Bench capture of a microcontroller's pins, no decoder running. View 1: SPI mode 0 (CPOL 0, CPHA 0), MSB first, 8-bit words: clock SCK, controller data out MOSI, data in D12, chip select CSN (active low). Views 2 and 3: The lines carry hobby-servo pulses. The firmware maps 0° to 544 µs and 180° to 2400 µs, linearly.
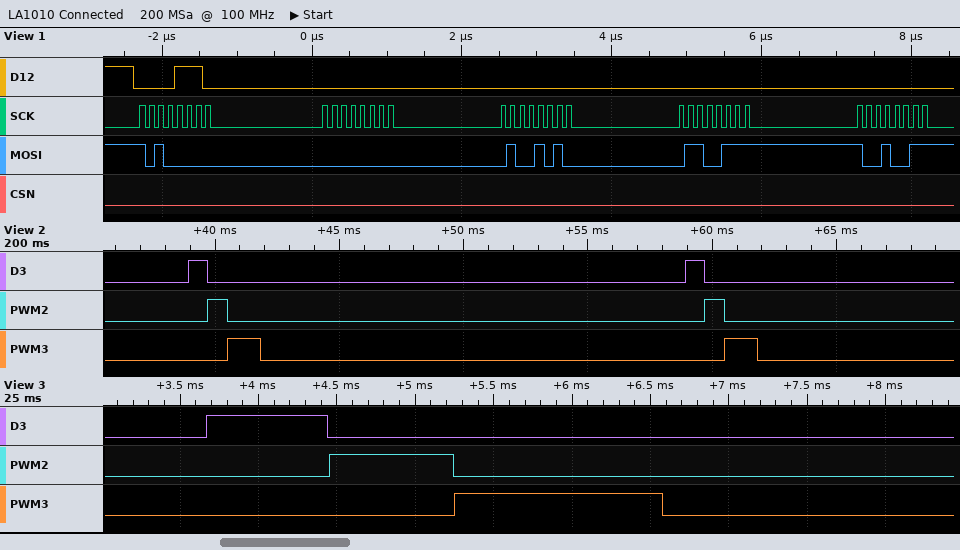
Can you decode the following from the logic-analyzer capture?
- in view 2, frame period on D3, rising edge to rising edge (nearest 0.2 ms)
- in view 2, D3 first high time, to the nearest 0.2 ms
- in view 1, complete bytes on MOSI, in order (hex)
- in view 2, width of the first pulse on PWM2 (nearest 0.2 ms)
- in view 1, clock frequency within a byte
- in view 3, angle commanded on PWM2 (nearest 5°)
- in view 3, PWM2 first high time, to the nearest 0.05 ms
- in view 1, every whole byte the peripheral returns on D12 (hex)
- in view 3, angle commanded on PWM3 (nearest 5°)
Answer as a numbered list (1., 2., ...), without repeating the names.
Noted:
1. 20.0 ms
2. 0.8 ms
3. A0 00 4A 67 93
4. 0.8 ms
5. 8 MHz
6. 25°
7. 0.80 ms
8. 0E 00 00 00 00
9. 75°
